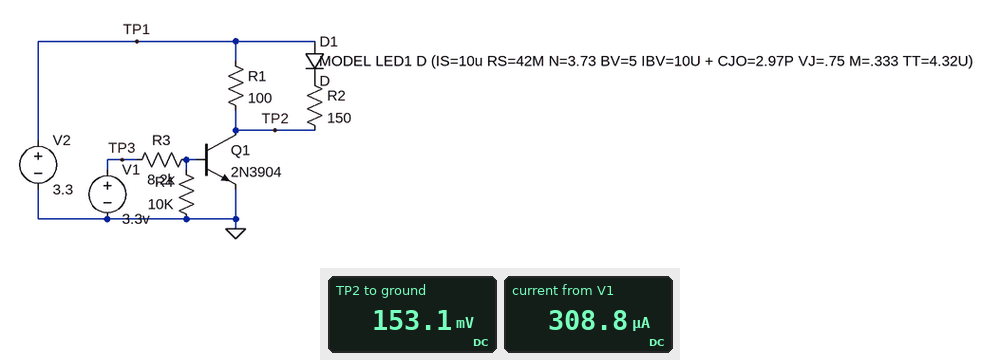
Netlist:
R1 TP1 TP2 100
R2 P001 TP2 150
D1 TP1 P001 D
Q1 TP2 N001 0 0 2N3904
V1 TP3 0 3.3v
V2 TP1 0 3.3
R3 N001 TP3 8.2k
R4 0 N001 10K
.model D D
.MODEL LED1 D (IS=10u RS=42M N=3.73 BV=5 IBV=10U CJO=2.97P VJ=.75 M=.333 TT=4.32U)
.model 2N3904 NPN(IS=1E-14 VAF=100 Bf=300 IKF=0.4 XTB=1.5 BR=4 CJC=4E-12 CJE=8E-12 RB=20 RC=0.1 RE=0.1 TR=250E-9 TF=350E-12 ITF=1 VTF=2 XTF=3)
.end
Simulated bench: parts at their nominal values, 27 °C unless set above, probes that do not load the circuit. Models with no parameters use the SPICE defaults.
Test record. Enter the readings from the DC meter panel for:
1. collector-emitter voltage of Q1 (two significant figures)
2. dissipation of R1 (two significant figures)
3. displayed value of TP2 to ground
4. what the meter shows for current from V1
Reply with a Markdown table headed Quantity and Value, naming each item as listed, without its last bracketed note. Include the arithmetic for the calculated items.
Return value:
| Quantity | Value |
|---|---|
| collector-emitter voltage of Q1 | 153.1 mV = 150 mV |
| dissipation of R1 | (3.3 V - 153.1 mV)^2 / 100 Ω = 99 mW |
| displayed value of TP2 to ground | 153.1 mV |
| what the meter shows for current from V1 | 308.8 µA |
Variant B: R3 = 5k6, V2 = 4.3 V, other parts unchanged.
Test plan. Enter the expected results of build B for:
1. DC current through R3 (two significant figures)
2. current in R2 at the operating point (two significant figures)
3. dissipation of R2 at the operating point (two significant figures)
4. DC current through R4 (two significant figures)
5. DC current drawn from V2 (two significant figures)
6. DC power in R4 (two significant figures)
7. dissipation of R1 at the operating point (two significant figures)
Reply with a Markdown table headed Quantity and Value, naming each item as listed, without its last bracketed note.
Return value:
| Quantity | Value |
|---|---|
| DC current through R3 | 450 µA |
| current in R2 at the operating point | 23 mA |
| dissipation of R2 at the operating point | 78 mW |
| DC current through R4 | 78 µA |
| DC current drawn from V2 | 64 mA |
| DC power in R4 | 61 µW |
| dissipation of R1 at the operating point | 170 mW |
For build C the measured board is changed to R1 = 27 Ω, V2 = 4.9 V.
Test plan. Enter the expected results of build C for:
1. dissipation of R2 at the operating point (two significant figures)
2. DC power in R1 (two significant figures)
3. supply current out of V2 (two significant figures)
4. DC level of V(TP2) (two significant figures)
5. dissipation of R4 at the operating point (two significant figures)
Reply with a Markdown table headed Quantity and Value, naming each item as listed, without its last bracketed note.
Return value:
| Quantity | Value |
|---|---|
| dissipation of R2 at the operating point | 4.5 mW |
| DC power in R1 | 85 mW |
| supply current out of V2 | 62 mA |
| DC level of V(TP2) | 3.4 V |
| dissipation of R4 at the operating point | 60 µW |
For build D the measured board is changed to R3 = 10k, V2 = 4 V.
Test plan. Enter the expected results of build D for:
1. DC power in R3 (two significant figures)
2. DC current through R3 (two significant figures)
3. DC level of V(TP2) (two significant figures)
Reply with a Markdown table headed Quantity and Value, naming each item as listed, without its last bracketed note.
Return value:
| Quantity | Value |
|---|---|
| DC power in R3 | 640 µW |
| DC current through R3 | 250 µA |
| DC level of V(TP2) | 860 mV |
